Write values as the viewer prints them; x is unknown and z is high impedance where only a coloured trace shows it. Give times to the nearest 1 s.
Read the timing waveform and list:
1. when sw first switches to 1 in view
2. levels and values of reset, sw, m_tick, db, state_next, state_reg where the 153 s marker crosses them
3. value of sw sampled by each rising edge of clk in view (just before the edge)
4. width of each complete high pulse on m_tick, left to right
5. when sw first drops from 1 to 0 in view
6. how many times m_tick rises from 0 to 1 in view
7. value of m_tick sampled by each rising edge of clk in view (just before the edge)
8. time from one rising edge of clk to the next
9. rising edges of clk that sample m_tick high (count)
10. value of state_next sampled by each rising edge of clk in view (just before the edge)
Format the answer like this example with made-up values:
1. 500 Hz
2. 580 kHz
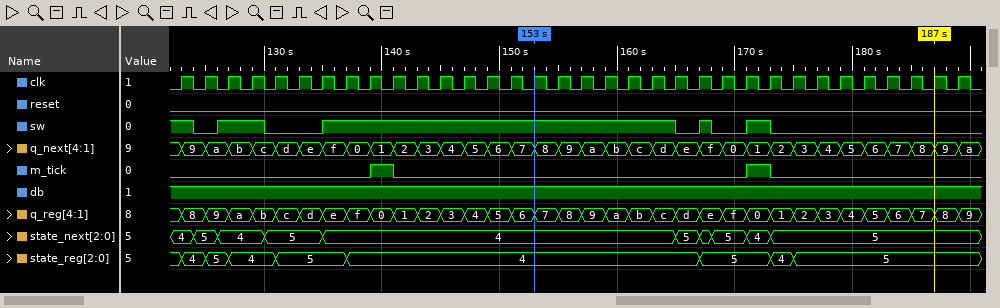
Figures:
1. 126 s
2. reset=0, sw=1, m_tick=0, db=1, state_next=4, state_reg=4
3. 1 0 1 1 0 0 0 1 1 1 1 1 1 1 1 1 1 1 1 1 1 1 0 0 0 1 0 0 0 0 0 0 0 0
4. 2 s, 2 s
5. 124 s
6. 2
7. 0 0 0 0 0 0 0 0 0 1 0 0 0 0 0 0 0 0 0 0 0 0 0 0 0 1 0 0 0 0 0 0 0 0
8. 2 s
9. 2
10. 4, 5, 4, 4, 5, 5, 5, 4, 4, 4, 4, 4, 4, 4, 4, 4, 4, 4, 4, 4, 4, 4, 5, 5, 5, 4, 5, 5, 5, 5, 5, 5, 5, 5
